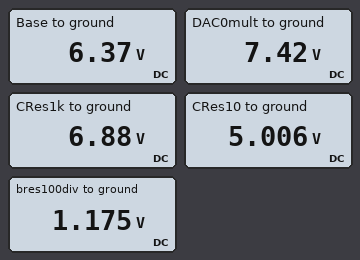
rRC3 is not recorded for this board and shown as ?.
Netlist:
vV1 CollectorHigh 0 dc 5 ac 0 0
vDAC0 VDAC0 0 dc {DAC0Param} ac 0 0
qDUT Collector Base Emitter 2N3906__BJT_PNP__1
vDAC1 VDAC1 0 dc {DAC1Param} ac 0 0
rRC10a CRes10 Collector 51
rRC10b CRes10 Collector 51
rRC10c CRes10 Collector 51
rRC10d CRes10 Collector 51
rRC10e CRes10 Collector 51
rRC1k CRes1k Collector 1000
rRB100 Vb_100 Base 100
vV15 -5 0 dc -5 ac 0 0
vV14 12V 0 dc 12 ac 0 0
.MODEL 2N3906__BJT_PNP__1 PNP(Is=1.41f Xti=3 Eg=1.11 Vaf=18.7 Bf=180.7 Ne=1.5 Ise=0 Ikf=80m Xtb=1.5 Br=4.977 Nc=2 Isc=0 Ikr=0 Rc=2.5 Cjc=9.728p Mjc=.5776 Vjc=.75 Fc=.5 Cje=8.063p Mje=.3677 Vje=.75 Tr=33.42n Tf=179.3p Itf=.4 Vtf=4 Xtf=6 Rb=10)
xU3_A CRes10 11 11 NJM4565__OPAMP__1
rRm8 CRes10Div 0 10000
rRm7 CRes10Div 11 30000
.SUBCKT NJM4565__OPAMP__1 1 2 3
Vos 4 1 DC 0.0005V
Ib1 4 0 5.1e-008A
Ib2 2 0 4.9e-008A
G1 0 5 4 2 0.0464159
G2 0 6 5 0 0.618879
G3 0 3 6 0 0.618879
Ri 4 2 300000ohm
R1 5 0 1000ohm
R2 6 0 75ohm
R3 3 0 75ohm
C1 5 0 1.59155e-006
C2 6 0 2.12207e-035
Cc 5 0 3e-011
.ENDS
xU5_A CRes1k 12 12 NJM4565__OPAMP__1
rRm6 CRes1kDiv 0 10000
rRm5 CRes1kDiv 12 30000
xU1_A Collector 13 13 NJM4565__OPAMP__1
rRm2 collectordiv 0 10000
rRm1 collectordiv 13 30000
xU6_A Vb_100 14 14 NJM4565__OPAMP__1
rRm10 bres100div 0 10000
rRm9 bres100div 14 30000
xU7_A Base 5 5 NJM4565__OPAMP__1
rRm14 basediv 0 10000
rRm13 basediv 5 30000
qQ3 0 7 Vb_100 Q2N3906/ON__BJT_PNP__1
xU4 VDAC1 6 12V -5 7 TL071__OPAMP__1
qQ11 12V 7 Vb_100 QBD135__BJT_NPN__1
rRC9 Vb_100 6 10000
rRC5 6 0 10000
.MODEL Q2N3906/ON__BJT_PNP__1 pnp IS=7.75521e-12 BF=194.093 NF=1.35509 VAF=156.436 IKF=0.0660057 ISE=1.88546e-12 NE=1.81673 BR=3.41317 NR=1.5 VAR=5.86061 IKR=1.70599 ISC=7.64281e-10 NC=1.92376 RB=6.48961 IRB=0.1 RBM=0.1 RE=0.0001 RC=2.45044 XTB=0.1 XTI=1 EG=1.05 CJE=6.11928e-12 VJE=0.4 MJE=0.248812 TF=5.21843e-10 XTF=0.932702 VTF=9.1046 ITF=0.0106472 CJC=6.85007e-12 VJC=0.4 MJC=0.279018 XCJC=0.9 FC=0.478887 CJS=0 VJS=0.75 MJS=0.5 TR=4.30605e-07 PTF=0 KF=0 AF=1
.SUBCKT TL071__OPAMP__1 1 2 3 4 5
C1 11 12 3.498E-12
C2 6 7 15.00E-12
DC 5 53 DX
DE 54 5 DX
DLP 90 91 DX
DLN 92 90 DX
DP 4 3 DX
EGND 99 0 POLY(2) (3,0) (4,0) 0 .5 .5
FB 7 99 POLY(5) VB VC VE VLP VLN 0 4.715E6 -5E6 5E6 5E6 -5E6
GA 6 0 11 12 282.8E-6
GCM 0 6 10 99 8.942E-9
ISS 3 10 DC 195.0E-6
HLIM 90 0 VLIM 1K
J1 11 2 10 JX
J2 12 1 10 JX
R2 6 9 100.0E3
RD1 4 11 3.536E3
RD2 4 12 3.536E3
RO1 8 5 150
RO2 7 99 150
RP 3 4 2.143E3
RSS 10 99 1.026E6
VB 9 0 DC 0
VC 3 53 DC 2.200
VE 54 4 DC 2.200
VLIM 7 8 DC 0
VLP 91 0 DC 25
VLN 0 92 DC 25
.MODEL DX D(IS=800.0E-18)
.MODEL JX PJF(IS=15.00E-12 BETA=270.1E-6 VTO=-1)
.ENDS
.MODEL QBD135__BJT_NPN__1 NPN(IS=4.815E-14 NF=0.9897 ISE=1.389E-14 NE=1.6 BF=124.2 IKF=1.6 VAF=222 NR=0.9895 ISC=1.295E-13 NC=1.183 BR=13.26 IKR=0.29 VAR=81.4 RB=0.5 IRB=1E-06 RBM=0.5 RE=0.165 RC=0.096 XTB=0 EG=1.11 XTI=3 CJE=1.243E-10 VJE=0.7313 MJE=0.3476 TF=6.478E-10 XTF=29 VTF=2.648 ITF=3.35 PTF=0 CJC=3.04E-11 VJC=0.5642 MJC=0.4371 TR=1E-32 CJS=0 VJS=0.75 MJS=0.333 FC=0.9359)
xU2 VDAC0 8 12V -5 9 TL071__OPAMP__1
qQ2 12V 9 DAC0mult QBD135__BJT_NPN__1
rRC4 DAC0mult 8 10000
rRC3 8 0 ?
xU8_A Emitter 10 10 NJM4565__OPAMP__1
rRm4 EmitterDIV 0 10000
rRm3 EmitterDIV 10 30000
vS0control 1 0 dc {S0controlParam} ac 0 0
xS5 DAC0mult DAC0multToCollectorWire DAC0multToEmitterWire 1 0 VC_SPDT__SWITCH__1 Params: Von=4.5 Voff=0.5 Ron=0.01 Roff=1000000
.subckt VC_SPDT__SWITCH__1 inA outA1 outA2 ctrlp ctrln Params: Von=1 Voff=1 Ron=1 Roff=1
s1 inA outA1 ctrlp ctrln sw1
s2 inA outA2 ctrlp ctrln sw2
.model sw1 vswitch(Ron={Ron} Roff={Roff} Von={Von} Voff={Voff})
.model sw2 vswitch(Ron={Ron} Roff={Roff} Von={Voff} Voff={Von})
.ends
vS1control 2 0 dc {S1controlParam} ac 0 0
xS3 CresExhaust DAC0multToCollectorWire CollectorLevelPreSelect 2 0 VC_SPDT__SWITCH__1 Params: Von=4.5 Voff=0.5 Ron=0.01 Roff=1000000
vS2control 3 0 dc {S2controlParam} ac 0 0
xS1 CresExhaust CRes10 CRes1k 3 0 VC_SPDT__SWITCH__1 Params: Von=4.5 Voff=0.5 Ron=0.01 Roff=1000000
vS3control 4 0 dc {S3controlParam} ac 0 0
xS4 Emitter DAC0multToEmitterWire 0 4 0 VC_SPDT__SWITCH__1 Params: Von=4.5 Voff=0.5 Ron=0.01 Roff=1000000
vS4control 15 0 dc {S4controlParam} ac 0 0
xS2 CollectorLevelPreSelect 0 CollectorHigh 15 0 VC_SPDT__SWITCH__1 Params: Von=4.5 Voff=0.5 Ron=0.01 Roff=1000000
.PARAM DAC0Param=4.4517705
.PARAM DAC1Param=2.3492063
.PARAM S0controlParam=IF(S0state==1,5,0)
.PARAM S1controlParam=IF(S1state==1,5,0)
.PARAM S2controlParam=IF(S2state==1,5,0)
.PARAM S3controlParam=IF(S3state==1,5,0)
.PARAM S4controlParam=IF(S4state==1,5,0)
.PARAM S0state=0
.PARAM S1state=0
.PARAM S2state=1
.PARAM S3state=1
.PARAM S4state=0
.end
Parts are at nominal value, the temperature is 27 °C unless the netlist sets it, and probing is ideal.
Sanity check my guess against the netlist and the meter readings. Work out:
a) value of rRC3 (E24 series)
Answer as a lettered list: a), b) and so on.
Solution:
a) 15 kΩ
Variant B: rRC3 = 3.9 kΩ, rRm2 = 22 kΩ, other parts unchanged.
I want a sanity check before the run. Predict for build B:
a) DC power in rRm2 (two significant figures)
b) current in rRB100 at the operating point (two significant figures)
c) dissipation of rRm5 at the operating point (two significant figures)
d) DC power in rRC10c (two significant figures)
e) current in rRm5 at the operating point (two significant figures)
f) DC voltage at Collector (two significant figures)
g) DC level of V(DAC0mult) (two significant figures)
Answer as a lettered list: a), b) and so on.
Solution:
a) 610 µW
b) 37 mA
c) 1.4 mW
d) 260 mW
e) 220 µA
f) 8.7 V
g) 9.6 V
